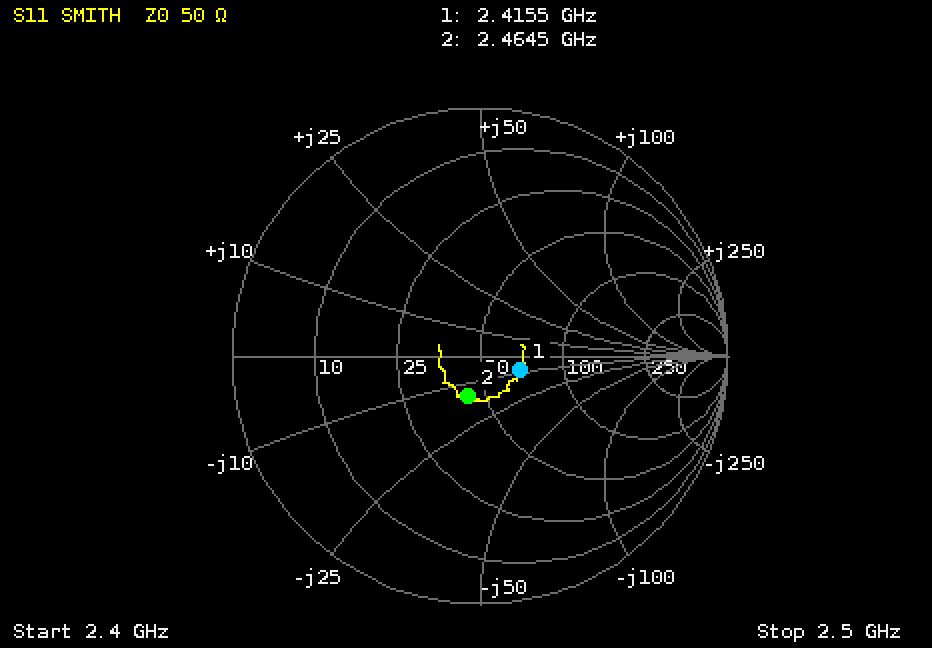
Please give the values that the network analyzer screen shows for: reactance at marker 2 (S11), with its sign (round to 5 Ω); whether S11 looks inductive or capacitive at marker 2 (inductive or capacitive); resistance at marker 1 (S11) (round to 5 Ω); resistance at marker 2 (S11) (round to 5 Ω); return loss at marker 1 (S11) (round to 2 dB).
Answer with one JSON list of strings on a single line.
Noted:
["-15 Ω", "capacitive", "70 Ω", "45 Ω", "16 dB"]
